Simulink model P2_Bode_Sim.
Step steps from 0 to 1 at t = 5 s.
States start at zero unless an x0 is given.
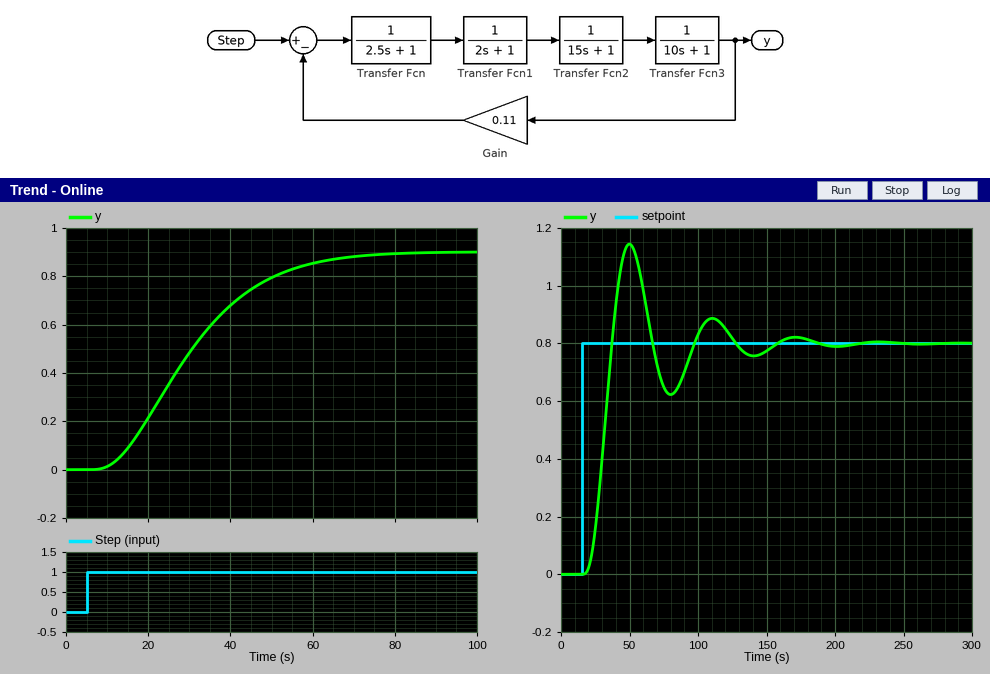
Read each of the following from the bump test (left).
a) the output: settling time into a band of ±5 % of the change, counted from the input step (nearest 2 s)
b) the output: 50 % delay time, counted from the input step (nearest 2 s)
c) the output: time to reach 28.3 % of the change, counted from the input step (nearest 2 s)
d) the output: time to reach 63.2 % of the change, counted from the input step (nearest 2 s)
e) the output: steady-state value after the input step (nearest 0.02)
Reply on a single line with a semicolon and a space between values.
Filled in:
56 s; 24 s; 16 s; 28 s; 0.90
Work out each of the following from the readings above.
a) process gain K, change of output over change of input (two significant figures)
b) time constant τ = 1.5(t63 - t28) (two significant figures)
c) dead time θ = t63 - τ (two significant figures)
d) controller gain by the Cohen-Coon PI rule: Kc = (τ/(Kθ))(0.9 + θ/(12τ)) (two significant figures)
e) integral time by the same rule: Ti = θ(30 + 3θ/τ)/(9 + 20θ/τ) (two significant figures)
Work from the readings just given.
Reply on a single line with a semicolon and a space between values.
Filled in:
0.90; 18 s; 10 s; 1.9; 16 s
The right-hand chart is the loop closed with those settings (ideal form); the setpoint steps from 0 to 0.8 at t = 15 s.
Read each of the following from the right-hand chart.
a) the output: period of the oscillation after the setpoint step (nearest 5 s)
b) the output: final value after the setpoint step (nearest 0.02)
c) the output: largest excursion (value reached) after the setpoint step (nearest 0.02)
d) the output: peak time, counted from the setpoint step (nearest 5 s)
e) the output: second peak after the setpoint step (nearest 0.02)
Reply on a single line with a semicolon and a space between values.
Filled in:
60 s; 0.80; 1.14; 35 s; 0.88
